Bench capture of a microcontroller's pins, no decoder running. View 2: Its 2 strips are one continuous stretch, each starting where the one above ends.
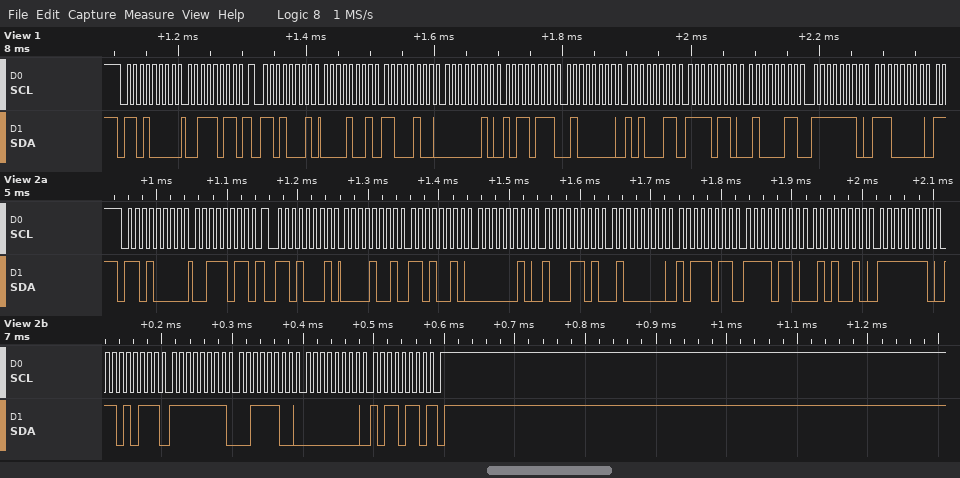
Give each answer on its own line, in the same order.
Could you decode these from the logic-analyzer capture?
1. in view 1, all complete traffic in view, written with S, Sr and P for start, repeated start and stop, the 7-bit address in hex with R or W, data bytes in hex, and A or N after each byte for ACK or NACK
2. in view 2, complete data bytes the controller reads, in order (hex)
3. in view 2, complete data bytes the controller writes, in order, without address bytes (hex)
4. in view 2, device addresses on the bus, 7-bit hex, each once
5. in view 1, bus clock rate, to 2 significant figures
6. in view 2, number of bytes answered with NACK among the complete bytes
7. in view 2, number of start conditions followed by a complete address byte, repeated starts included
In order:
S 68W A 3B A Sr 68R A 09 A C4 A 02 A B7 A 40 A A3 A F6 A 43 A FE A E0 A
09 D2 02 8D 40 BB F6 52 FE D7 FF 3C 00 B6
3B
0x68
100 kHz
1
2
